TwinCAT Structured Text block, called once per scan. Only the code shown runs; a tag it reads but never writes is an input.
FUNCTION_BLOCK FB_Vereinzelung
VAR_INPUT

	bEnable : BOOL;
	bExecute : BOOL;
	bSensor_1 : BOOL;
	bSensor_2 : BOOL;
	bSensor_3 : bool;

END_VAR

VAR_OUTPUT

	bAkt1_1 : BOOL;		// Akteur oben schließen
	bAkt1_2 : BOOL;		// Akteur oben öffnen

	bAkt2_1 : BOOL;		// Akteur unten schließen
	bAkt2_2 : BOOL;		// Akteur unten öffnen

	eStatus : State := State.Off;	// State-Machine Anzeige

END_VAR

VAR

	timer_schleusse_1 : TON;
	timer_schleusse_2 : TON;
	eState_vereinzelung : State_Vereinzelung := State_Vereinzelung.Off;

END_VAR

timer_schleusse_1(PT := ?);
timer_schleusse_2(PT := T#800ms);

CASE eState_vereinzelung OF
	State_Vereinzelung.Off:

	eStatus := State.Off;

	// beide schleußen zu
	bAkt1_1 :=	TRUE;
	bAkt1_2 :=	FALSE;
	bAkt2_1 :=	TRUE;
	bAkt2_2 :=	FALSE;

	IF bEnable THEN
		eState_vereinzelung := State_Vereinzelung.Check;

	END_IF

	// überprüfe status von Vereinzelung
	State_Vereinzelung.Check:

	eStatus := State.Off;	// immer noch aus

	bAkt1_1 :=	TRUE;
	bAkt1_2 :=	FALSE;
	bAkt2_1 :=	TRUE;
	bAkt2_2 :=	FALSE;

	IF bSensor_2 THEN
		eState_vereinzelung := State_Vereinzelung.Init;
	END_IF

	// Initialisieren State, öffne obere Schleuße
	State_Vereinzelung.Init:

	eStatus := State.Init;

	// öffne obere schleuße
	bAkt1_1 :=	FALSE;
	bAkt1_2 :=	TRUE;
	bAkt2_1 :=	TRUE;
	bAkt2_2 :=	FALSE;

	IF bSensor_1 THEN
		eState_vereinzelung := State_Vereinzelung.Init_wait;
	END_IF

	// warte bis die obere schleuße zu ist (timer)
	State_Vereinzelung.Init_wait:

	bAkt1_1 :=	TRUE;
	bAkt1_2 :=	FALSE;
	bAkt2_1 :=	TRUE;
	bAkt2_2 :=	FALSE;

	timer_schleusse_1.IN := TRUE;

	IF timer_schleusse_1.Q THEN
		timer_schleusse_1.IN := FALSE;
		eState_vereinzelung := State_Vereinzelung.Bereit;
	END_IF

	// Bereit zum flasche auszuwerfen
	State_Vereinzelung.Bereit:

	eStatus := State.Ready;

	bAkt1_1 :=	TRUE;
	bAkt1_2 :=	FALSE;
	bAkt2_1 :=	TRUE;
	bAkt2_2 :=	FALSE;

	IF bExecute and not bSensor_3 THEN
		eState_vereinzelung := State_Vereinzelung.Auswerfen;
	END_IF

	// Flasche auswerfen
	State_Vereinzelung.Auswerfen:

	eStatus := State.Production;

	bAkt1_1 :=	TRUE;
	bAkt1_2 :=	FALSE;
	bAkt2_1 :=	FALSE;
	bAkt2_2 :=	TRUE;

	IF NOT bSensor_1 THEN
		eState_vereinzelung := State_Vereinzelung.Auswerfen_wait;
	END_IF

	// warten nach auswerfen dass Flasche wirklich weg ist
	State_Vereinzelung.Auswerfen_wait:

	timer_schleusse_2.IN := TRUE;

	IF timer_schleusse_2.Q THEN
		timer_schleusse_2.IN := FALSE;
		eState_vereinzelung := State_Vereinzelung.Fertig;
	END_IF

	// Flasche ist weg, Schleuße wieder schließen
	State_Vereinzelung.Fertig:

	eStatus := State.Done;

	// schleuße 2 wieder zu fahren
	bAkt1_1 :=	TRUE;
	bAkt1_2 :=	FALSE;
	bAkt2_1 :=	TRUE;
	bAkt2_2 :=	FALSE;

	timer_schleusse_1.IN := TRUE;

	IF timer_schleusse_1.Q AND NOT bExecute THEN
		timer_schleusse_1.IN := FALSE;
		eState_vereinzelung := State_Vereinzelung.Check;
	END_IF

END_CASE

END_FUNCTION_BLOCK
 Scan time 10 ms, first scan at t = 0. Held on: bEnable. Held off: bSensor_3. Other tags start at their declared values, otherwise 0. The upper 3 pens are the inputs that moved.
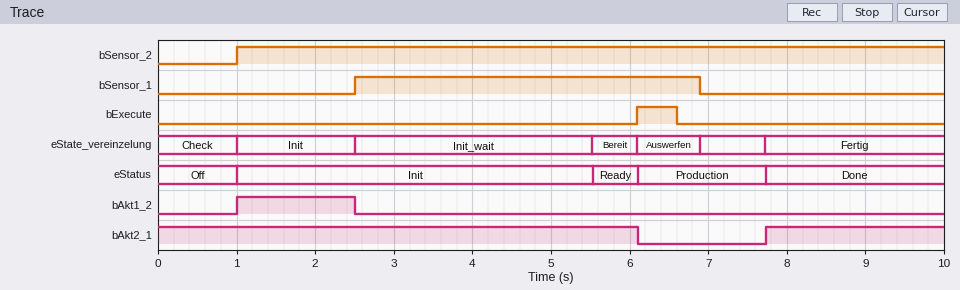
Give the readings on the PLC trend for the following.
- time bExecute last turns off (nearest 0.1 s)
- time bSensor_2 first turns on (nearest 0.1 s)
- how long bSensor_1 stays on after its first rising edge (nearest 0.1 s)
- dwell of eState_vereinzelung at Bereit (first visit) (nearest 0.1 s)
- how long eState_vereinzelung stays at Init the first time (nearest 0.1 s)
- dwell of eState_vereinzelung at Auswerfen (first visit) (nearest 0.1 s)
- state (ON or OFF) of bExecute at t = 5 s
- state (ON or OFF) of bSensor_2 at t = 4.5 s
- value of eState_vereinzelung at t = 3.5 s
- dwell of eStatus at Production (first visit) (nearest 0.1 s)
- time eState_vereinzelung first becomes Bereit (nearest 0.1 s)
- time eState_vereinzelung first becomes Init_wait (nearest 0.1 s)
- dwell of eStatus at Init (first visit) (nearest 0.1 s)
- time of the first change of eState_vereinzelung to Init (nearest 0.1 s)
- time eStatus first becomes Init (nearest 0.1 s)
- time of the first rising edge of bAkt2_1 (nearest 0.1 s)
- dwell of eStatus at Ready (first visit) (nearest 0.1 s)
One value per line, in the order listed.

6.6 s
1.0 s
4.4 s
0.6 s
1.5 s
0.8 s
OFF
ON
Init_wait
1.6 s
5.5 s
2.5 s
4.5 s
1.0 s
1.0 s
7.7 s
0.6 s
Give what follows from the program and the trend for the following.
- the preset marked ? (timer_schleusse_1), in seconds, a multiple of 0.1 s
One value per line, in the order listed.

3.0 s
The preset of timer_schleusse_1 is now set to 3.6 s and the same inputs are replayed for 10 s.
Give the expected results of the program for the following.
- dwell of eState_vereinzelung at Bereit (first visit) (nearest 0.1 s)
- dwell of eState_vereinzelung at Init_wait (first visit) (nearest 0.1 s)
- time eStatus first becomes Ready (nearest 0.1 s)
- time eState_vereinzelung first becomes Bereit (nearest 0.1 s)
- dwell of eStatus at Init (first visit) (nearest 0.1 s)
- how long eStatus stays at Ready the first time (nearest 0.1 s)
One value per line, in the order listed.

0.0 s
3.6 s
6.1 s
6.1 s
5.1 s
0.0 s
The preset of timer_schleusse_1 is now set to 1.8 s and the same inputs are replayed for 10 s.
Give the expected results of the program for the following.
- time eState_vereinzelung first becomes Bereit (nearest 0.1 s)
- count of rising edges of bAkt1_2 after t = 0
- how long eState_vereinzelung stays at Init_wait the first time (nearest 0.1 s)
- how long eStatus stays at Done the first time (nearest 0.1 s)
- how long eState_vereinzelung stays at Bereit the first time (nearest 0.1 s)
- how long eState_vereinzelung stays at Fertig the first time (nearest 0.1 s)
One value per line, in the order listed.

4.3 s
2
1.8 s
1.8 s
1.8 s
1.8 s
